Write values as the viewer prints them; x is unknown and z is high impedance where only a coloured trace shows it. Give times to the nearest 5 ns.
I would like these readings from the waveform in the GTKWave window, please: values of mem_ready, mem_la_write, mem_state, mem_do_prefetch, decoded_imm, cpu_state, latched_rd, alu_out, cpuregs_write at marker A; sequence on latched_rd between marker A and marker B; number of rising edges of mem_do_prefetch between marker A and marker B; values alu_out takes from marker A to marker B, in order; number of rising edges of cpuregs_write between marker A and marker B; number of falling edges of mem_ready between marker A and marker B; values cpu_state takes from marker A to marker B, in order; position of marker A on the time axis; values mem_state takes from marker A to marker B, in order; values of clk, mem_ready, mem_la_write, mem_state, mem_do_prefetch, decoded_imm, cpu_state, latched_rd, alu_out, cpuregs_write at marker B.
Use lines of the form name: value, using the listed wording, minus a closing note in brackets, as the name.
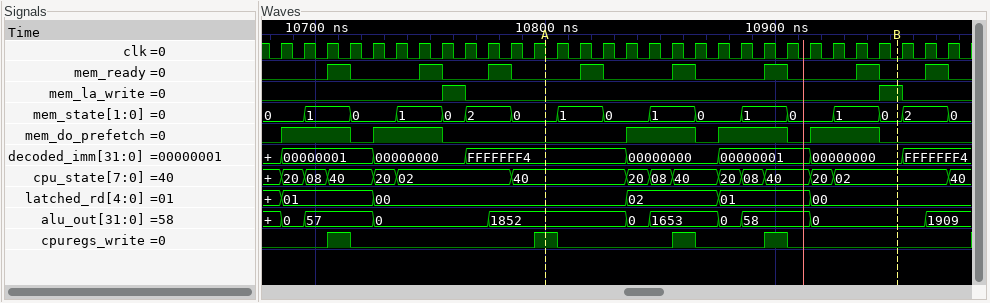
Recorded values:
values of mem_ready, mem_la_write, mem_state, mem_do_prefetch, decoded_imm, cpu_state, latched_rd, alu_out, cpuregs_write at marker A: mem_ready=0, mem_la_write=0, mem_state=0, mem_do_prefetch=0, decoded_imm=FFFFFFF4, cpu_state=40, latched_rd=00, alu_out=1852, cpuregs_write=1
sequence on latched_rd between marker A and marker B: 00, 02, 01, 00
number of rising edges of mem_do_prefetch between marker A and marker B: 3
values alu_out takes from marker A to marker B, in order: 1852, 0, 1653, 0, 58, 0
number of rising edges of cpuregs_write between marker A and marker B: 2
number of falling edges of mem_ready between marker A and marker B: 4
values cpu_state takes from marker A to marker B, in order: 40, 20, 08, 40, 20, 08, 40, 20, 02
position of marker A on the time axis: 10800 ns
values mem_state takes from marker A to marker B, in order: 0, 1, 0, 1, 0, 1, 0, 1, 0
values of clk, mem_ready, mem_la_write, mem_state, mem_do_prefetch, decoded_imm, cpu_state, latched_rd, alu_out, cpuregs_write at marker B: clk=0, mem_ready=0, mem_la_write=1, mem_state=0, mem_do_prefetch=0, decoded_imm=00000000, cpu_state=02, latched_rd=00, alu_out=0, cpuregs_write=0
